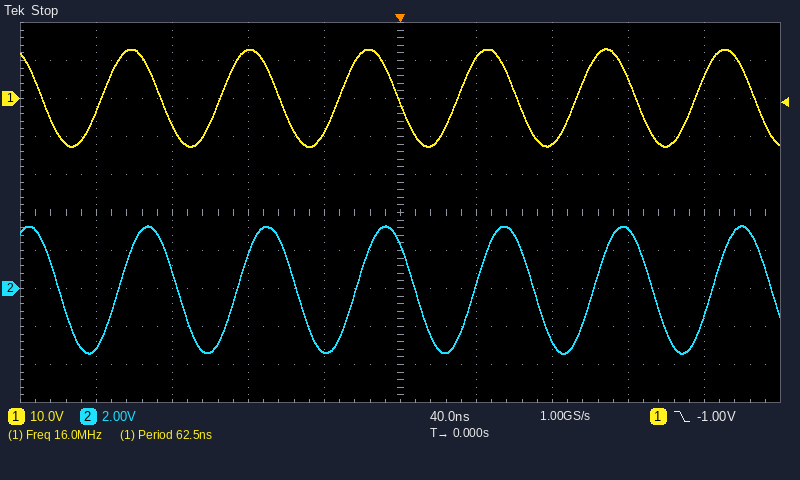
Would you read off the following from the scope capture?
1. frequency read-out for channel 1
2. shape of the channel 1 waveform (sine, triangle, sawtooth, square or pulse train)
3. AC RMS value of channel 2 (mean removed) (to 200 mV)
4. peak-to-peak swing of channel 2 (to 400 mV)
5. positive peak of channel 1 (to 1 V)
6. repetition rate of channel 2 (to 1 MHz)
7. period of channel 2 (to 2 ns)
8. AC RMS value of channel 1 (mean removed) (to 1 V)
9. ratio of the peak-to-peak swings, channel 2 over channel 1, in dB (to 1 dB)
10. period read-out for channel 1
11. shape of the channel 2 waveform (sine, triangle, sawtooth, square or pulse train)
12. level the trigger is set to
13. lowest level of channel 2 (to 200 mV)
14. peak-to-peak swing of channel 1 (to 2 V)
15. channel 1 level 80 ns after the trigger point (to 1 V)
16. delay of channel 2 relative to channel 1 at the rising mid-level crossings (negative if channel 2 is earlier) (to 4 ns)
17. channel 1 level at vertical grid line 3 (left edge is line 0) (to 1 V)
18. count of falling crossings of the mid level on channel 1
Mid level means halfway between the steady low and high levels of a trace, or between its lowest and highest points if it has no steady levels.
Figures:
16.0 MHz
sine
2.4 V
6.8 V
13 V
16 MHz
62 ns
9 V
-12 dB
62.5 ns
sine
-1.00 V
-3.4 V
26 V
-12 V
+8 ns
13 V
7
